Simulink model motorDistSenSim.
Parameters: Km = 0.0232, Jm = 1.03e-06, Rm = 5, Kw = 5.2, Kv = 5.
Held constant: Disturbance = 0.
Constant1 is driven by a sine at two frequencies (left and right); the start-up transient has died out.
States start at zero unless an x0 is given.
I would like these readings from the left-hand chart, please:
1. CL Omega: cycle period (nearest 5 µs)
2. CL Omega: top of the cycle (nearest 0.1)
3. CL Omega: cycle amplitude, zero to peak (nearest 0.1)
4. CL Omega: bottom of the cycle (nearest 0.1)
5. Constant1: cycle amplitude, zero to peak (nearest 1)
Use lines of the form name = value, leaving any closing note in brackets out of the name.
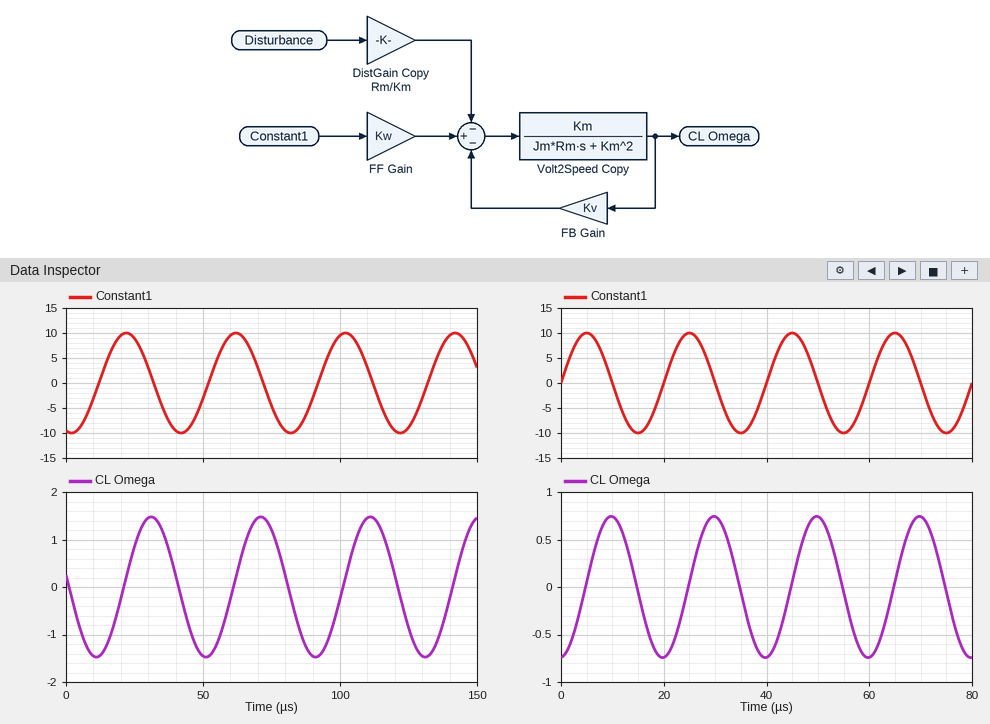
CL Omega: cycle period = 40 µs
CL Omega: top of the cycle = 1.5
CL Omega: cycle amplitude, zero to peak = 1.5
CL Omega: bottom of the cycle = -1.5
Constant1: cycle amplitude, zero to peak = 10
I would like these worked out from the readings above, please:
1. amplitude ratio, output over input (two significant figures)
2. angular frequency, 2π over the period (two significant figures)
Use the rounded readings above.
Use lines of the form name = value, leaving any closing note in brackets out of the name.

amplitude ratio, output over input = 0.15
angular frequency, 2π over the period = 0.16 rad/µs
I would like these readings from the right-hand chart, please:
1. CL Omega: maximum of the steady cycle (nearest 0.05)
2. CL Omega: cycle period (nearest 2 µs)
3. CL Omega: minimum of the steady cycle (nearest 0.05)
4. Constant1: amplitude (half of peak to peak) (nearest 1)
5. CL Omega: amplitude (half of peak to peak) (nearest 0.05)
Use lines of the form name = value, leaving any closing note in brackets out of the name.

CL Omega: maximum of the steady cycle = 0.75
CL Omega: cycle period = 20 µs
CL Omega: minimum of the steady cycle = -0.75
Constant1: amplitude (half of peak to peak) = 10
CL Omega: amplitude (half of peak to peak) = 0.75
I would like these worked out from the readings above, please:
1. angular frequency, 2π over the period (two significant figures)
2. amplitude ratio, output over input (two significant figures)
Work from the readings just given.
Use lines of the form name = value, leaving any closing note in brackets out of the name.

angular frequency, 2π over the period = 0.31 rad/µs
amplitude ratio, output over input = 0.075
